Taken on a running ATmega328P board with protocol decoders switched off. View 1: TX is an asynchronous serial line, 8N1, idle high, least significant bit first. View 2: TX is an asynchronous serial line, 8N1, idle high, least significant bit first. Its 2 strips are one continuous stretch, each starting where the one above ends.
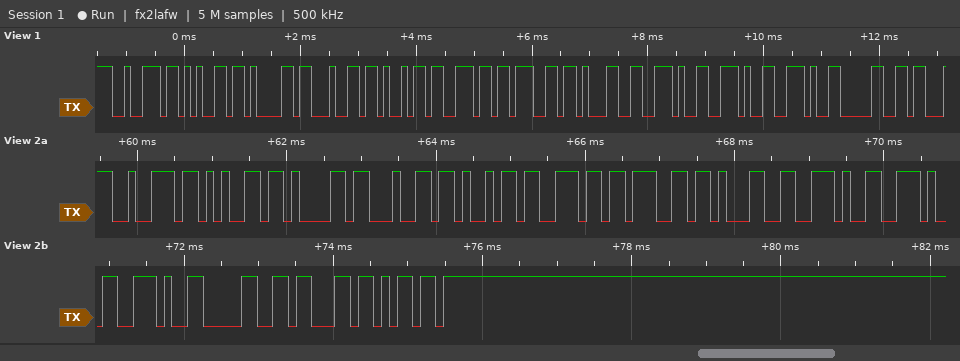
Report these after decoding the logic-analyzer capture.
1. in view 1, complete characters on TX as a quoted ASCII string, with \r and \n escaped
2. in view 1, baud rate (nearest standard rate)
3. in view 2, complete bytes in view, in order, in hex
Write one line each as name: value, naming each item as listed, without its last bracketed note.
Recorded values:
in view 1, complete characters on TX as a quoted ASCII string, with \r and \n escaped: "reading1...0"
in view 1, baud rate: 9600 baud
in view 2, complete bytes in view, in order, in hex: 0x72 0x65 0x61 0x64 0x69 0x6E 0x67 0x31 0x2E 0x2E 0x2E 0x30 0x63 0x6D
